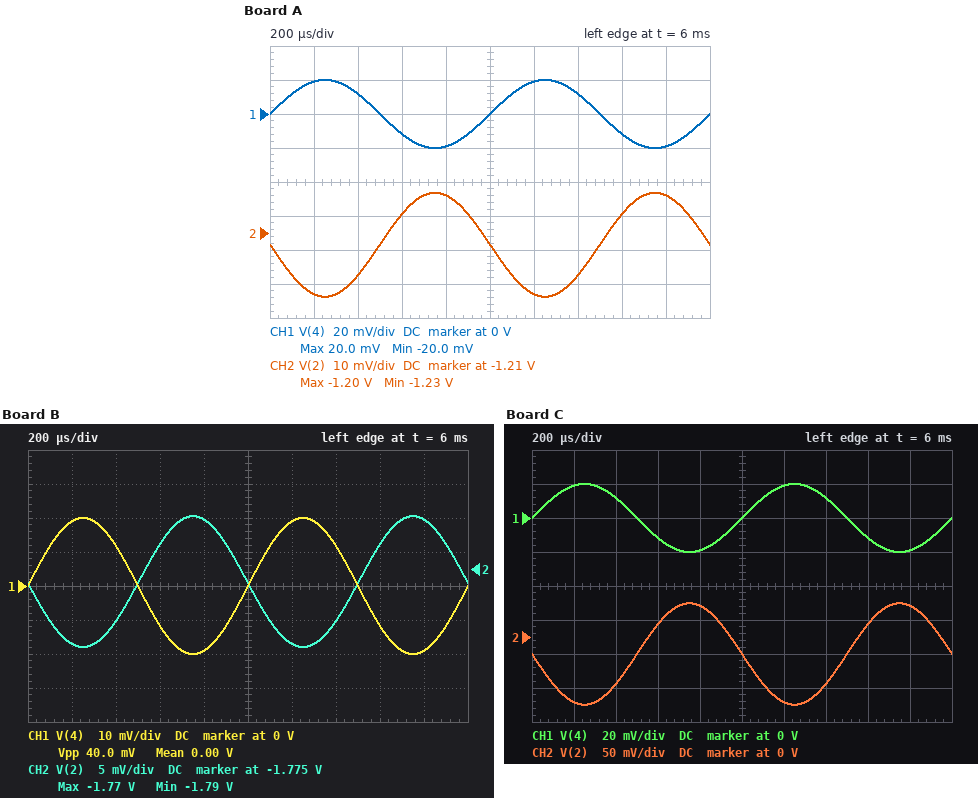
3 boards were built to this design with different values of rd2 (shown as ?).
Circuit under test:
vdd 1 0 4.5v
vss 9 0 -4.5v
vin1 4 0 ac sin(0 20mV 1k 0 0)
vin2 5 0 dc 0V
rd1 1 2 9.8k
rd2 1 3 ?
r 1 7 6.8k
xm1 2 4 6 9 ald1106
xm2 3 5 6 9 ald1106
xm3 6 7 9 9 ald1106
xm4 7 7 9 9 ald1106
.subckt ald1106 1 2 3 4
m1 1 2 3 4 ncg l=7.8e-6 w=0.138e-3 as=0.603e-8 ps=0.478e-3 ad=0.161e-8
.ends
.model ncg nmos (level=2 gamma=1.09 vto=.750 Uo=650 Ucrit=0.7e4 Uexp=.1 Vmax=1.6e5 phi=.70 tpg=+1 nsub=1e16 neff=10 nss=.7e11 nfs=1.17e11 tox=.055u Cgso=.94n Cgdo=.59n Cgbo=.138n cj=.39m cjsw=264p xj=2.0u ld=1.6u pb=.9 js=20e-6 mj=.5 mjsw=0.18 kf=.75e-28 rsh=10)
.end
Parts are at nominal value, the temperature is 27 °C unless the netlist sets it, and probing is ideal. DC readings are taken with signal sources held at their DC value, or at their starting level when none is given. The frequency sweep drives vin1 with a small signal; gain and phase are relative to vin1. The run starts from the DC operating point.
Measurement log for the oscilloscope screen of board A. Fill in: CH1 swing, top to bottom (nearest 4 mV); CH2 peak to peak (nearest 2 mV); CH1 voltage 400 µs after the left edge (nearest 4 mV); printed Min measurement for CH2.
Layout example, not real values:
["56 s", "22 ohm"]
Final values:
["40 mV", "30 mV", "12 mV", "-1.23 V"]
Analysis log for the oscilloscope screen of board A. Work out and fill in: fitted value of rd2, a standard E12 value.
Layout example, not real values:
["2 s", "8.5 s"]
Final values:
["18 kΩ"]
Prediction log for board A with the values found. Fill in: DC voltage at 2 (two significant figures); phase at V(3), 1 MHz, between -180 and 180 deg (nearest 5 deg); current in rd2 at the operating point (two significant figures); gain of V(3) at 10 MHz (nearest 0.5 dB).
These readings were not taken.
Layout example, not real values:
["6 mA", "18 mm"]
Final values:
["-1.2 V", "0 deg", "370 µA", "0 dB"]
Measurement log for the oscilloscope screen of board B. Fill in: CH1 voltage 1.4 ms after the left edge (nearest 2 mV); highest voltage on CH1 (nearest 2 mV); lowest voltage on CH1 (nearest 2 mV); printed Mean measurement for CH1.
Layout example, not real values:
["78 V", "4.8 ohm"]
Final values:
["12 mV", "20 mV", "-20 mV", "0.00 V"]
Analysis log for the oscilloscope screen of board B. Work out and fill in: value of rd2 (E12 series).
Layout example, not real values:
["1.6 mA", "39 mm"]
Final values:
["22 kΩ"]
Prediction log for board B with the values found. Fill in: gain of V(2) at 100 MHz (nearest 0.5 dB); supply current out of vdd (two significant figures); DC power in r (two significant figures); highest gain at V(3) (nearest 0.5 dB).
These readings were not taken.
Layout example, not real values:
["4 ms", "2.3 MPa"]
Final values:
["2.5 dB", "1.9 mA", "6.4 mW", "-3.5 dB"]
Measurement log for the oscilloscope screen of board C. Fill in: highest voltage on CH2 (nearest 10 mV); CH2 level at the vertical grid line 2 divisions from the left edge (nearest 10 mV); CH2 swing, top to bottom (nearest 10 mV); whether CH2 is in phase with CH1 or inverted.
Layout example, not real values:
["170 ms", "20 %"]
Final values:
["50 mV", "-70 mV", "150 mV", "inverted"]
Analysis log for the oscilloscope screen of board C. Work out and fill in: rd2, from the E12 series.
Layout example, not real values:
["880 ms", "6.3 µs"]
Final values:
["3.3 kΩ"]
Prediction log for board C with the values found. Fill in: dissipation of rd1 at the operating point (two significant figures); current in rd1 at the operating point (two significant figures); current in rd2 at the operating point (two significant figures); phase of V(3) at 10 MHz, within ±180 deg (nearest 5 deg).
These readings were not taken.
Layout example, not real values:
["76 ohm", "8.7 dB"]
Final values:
["2.1 mW", "460 µA", "500 µA", "-10 deg"]
